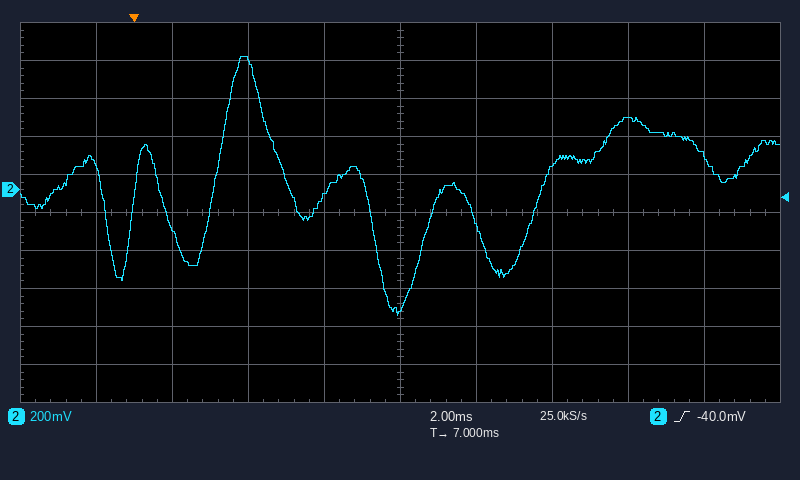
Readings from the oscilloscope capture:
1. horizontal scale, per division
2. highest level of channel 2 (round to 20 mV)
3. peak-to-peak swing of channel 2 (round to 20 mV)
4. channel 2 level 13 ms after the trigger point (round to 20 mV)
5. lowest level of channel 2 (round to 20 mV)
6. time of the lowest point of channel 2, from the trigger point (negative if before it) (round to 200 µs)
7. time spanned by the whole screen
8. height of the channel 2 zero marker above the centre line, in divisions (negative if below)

2 ms
700 mV
1.36 V
380 mV
-660 mV
+7.0 ms
20 ms
+0.6 div
